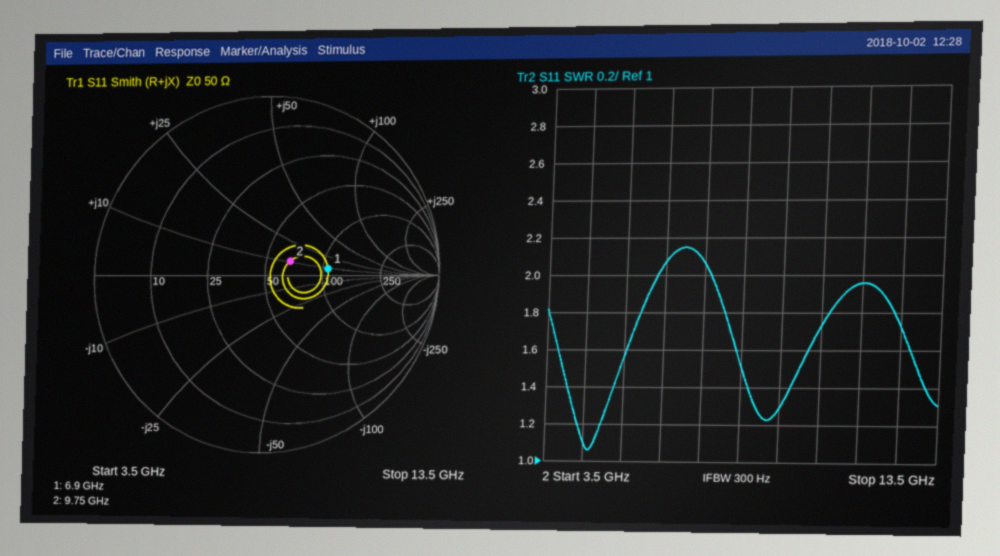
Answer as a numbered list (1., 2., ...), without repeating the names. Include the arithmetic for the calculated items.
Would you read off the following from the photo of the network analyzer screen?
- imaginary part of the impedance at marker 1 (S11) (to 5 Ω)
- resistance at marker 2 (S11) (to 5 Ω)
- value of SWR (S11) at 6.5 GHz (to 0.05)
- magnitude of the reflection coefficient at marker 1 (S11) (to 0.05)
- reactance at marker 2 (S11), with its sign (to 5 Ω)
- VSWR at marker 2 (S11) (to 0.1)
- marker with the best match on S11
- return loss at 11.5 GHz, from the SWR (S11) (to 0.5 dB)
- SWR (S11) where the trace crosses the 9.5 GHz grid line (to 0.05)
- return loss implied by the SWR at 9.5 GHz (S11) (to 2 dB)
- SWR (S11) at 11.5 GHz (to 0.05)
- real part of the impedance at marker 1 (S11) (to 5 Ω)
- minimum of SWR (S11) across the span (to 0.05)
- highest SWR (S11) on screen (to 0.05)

1. +10 Ω
2. 65 Ω
3. 2.05
4. 0.35
5. +10 Ω
6. 1.4
7. marker 2
8. −20 log10((1.95 − 1)/(1.95 + 1)) ≈ 9.84 dB, so 10.0 dB to the nearest 0.5 dB
9. 1.30
10. −20 log10((1.3 − 1)/(1.3 + 1)) ≈ 18 dB
11. 1.95
12. 105 Ω
13. 1.05
14. 2.15
